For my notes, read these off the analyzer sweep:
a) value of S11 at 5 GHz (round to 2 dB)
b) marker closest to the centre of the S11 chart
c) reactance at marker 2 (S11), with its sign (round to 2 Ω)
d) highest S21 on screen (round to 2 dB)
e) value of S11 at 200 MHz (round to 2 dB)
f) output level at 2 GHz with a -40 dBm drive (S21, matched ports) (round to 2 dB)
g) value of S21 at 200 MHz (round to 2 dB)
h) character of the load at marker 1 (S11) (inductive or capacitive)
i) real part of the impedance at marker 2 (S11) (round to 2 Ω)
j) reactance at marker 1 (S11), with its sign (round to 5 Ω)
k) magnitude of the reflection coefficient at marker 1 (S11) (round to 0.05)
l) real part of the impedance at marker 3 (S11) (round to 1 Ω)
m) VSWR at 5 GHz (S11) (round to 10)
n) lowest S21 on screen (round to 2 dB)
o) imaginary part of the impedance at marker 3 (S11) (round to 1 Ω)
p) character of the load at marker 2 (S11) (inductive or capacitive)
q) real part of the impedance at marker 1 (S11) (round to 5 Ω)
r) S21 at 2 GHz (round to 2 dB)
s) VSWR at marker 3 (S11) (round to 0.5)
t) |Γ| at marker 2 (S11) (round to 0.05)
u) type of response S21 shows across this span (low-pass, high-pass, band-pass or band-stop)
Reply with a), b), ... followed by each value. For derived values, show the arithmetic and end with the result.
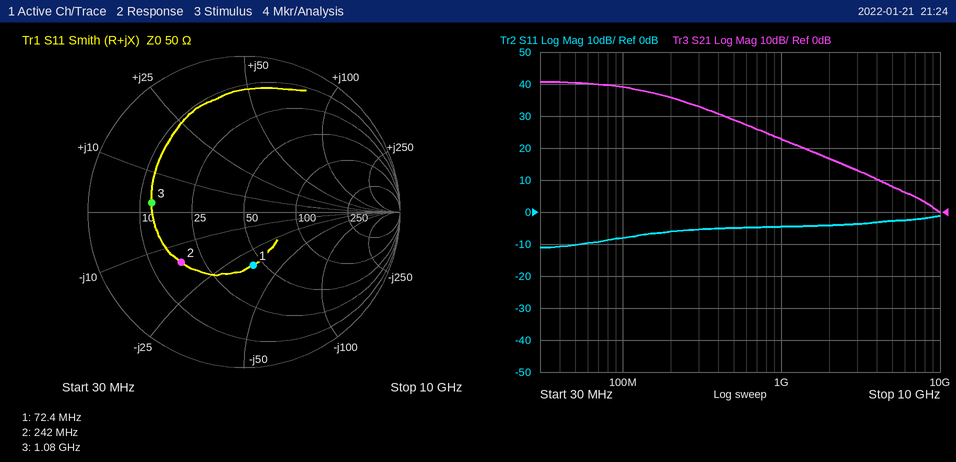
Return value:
a) -2 dB
b) marker 1
c) -16 Ω
d) 40 dB
e) -6 dB
f) -40 dBm + (16 dB) = -24 dBm
g) 36 dB
h) capacitive
i) 18 Ω
j) -35 Ω
k) 0.35
l) 13 Ω
m) |Γ| = 10^(-2/20) = 0.7943; VSWR = (1 + 0.7943)/(1 − 0.7943) ≈ 8.72, so 10 to the nearest 10
n) 0 dB
o) +2 Ω
p) capacitive
q) 45 Ω
r) 16 dB
s) 4.0
t) 0.50
u) low-pass
